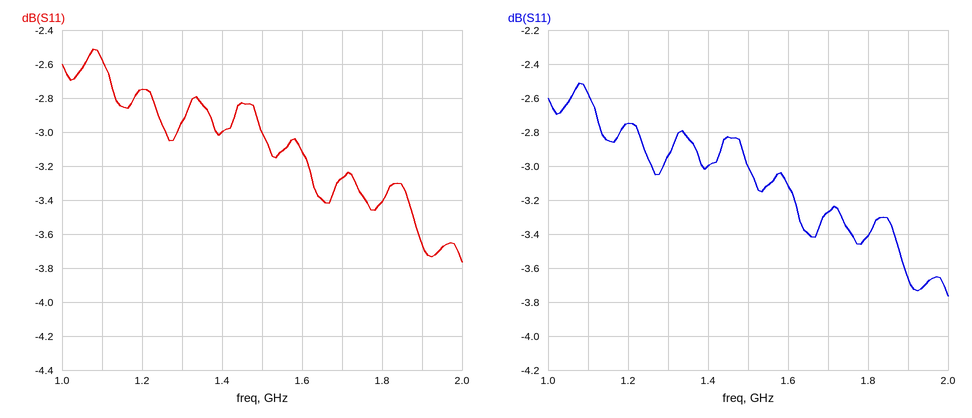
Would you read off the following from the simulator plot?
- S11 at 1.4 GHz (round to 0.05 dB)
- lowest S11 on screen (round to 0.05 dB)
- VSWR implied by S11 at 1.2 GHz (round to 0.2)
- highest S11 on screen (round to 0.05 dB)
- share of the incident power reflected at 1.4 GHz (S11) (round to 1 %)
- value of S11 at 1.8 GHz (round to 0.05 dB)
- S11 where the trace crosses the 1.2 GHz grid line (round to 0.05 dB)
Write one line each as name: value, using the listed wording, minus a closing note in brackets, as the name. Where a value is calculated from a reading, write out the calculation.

S11 at 1.4 GHz: -3.00 dB
lowest S11 on screen: -3.75 dB
VSWR implied by S11 at 1.2 GHz: |Γ| = 10^(-2.75/20) = 0.7286; VSWR = (1 + 0.7286)/(1 − 0.7286) ≈ 6.4
highest S11 on screen: -2.50 dB
share of the incident power reflected at 1.4 GHz (S11): 10^(-3/10) ≈ 50 %
value of S11 at 1.8 GHz: -3.40 dB
S11 where the trace crosses the 1.2 GHz grid line: -2.75 dB
